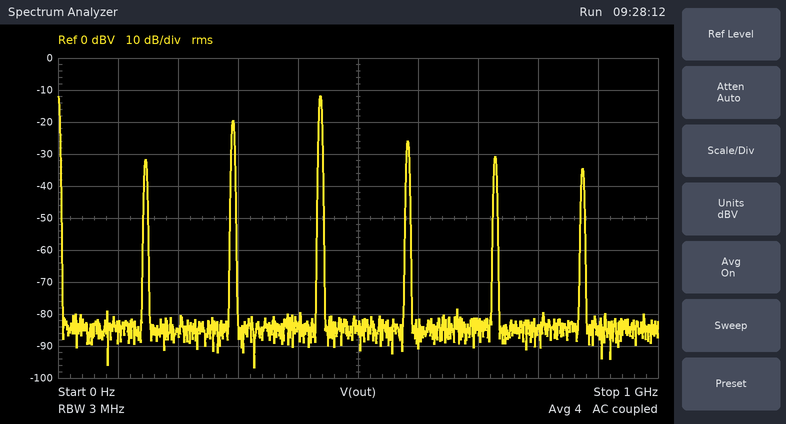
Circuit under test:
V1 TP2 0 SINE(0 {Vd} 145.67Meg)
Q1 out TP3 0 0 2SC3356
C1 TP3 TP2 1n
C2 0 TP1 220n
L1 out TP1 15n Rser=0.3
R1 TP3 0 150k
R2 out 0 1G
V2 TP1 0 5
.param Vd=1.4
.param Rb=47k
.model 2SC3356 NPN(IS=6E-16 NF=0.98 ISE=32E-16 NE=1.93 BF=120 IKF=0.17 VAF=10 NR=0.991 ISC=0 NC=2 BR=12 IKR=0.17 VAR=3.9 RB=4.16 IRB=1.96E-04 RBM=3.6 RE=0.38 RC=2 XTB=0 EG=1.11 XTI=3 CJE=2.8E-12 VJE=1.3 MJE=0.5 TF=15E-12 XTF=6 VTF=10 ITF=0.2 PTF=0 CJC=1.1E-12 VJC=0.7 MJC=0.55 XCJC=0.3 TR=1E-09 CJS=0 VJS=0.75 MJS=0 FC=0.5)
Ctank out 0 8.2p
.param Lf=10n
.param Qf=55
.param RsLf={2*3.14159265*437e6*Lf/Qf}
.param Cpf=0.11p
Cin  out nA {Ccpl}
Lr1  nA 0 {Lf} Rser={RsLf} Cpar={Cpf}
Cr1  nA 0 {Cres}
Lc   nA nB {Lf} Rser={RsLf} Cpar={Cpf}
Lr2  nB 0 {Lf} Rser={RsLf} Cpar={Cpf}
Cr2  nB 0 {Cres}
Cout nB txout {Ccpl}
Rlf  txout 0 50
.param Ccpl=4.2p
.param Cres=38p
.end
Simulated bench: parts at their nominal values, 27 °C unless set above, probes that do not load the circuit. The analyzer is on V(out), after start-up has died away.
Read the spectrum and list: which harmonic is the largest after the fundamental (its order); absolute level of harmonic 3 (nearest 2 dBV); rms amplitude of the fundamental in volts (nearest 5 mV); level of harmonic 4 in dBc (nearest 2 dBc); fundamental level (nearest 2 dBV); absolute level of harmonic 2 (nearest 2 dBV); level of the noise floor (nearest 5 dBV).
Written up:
3
-12 dBV
25 mV
6 dBc
-32 dBV
-20 dBV
-85 dBV
